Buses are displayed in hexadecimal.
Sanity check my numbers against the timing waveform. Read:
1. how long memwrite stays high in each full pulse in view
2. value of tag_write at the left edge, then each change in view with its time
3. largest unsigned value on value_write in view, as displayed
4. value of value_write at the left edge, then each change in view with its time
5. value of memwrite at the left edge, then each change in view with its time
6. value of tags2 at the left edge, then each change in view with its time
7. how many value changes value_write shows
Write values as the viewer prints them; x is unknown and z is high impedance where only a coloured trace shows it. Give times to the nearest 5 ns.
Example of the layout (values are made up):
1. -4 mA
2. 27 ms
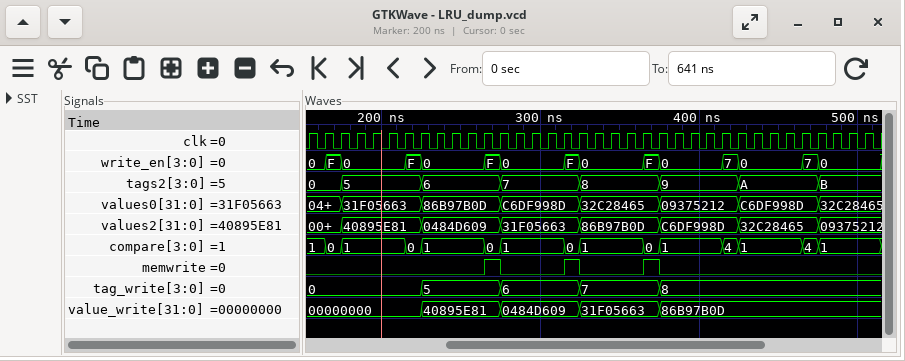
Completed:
1. 10 ns, 10 ns, 10 ns
2. 0, 5 at 225 ns, 6 at 275 ns, 7 at 325 ns, 8 at 375 ns
3. 86B97B0D
4. 00000000, 40895E81 at 225 ns, 0484D609 at 275 ns, 31F05663 at 325 ns, 86B97B0D at 375 ns
5. 0, 1 at 265 ns, 0 at 275 ns, 1 at 315 ns, 0 at 325 ns, 1 at 365 ns, 0 at 375 ns
6. 0, 5 at 175 ns, 6 at 225 ns, 7 at 275 ns, 8 at 325 ns, 9 at 375 ns, A at 425 ns, B at 475 ns
7. 4
